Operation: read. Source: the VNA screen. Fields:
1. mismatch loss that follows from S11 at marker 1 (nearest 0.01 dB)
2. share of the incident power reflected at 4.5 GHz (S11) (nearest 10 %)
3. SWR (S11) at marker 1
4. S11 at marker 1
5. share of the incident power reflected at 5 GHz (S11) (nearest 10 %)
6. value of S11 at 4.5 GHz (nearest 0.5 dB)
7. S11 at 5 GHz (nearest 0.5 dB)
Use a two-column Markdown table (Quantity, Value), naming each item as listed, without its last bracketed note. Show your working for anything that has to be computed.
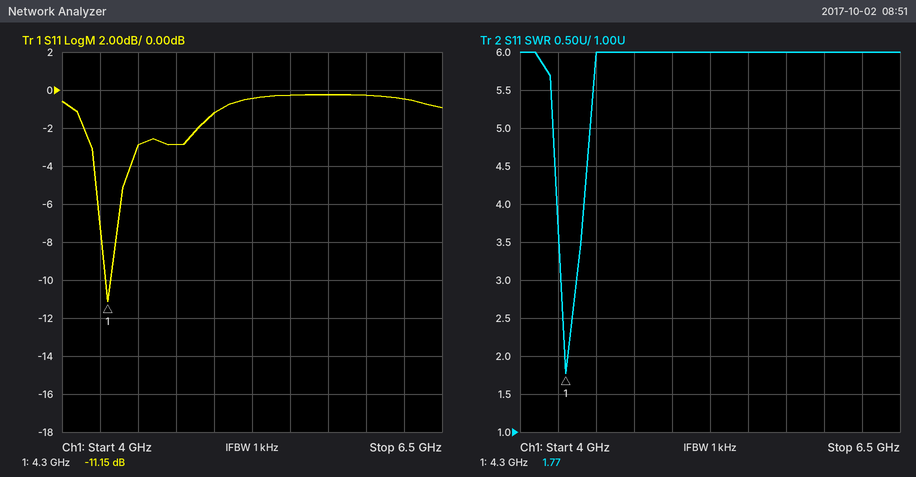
| Quantity | Value |
|---|---|
| mismatch loss that follows from S11 at marker 1 | −10 log10(1 − 10^(-11.15/10)) ≈ 0.35 dB |
| share of the incident power reflected at 4.5 GHz (S11) | 10^(-3/10) ≈ 50 % |
| SWR (S11) at marker 1 | 1.77 |
| S11 at marker 1 | -11.15 dB |
| share of the incident power reflected at 5 GHz (S11) | 10^(-1/10) ≈ 79.4 %, so 80 % to the nearest 10 % |
| value of S11 at 4.5 GHz | -3.0 dB |
| S11 at 5 GHz | -1.0 dB |
